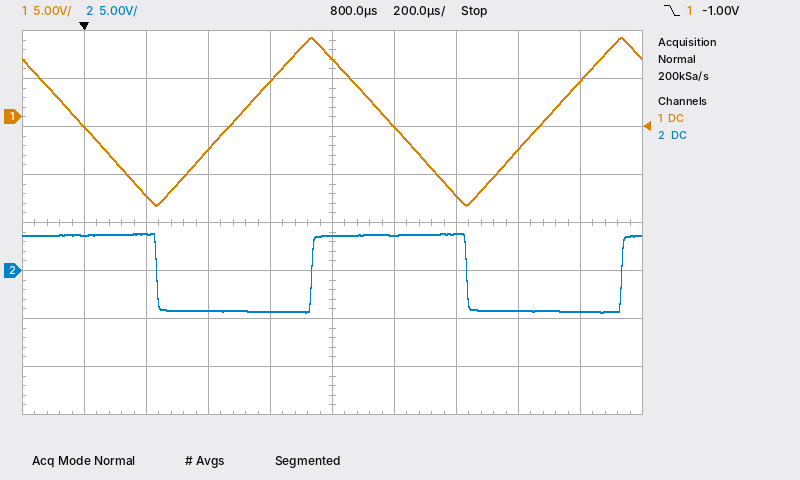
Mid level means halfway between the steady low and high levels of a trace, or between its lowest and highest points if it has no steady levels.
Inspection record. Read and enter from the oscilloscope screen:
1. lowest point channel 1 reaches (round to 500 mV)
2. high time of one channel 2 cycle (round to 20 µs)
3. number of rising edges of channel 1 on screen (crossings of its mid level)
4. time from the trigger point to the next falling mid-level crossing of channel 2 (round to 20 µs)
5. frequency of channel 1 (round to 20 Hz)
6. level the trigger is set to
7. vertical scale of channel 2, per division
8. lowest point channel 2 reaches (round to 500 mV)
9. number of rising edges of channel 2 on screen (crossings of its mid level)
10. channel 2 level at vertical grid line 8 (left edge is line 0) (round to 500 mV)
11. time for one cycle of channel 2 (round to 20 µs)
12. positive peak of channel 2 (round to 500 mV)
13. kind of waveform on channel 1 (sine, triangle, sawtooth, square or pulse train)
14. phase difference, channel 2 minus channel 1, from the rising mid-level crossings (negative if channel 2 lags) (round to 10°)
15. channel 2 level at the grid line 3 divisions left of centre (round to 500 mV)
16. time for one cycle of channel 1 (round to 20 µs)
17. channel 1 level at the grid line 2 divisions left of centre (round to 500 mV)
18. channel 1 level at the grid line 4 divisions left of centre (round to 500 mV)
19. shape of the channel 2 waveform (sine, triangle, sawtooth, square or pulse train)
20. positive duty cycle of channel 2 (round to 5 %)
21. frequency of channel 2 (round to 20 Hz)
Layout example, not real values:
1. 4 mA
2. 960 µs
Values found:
1. -9.0 V
2. 500 µs
3. 2
4. 240 µs
5. 1.00 kHz
6. -1.00 V
7. 5 V
8. -4.5 V
9. 2
10. -4.0 V
11. 1.00 ms
12. 4.0 V
13. triangle
14. -90°
15. 4.0 V
16. 1.00 ms
17. -3.5 V
18. -1.0 V
19. square
20. 50 %
21. 1.00 kHz
